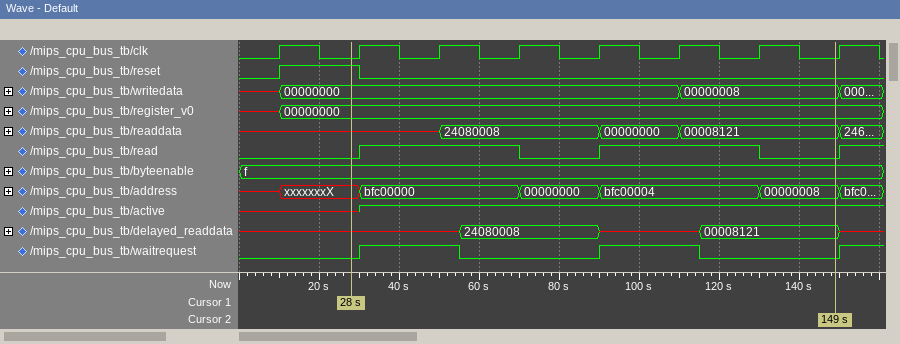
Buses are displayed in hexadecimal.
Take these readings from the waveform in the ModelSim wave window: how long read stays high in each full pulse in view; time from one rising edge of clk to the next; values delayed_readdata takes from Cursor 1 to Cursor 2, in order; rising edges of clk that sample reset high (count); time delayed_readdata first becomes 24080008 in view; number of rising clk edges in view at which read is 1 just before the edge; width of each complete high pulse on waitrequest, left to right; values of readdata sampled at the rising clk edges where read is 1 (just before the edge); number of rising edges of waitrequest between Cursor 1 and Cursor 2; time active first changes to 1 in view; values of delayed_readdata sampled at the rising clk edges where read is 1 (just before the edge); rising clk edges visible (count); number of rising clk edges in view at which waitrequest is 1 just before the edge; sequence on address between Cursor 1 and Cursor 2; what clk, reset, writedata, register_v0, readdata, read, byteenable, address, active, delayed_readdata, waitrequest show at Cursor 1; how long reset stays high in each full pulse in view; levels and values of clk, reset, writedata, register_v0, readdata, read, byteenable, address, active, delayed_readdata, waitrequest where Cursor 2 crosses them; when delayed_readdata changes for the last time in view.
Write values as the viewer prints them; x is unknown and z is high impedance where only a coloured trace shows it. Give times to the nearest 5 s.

40 s, 40 s
20 s
x, 24080008, x, 00008121
1
55 s
4
25 s, 25 s
x, 24080008, 00000000, 00008121
2
30 s
x, 24080008, x, 00008121
8
2
xxxxxxxX, bfc00000, 00000000, bfc00004, 00000008
clk=0, reset=1, writedata=00000000, register_v0=00000000, readdata=x, read=0, byteenable=f, address=xxxxxxxX, active=x, delayed_readdata=x, waitrequest=0
20 s
clk=0, reset=0, writedata=00000008, register_v0=00000000, readdata=00008121, read=0, byteenable=f, address=00000008, active=1, delayed_readdata=00008121, waitrequest=0
150 s
